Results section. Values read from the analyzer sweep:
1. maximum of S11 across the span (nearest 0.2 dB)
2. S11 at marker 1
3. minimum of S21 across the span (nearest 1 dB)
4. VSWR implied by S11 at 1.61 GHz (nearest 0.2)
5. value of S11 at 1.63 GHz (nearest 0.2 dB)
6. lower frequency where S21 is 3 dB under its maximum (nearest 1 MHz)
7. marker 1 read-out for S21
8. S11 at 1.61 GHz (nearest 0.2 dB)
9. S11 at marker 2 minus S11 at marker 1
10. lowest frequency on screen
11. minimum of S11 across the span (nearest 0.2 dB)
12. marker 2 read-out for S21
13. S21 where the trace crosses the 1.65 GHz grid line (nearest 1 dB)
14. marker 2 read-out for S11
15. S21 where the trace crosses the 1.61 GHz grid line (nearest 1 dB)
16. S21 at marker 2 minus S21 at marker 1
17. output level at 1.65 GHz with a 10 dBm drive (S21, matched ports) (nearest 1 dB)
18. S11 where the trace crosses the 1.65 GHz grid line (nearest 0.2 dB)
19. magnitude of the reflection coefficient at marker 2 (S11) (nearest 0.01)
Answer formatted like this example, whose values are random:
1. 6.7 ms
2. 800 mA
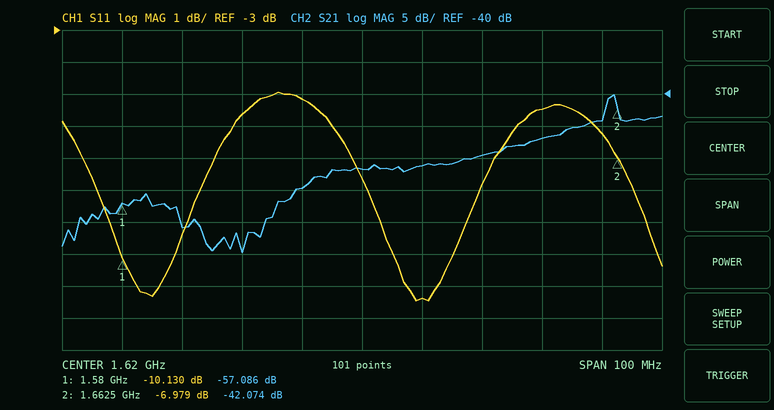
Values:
1. -5.0 dB
2. -10.130 dB
3. -65 dB
4. 3.4
5. -11.4 dB
6. 1.660 GHz
7. -57.086 dB
8. -5.2 dB
9. 3.151 dB
10. 1.57 GHz
11. -11.4 dB
12. -42.074 dB
13. -47 dB
14. -6.979 dB
15. -55 dB
16. 15.012 dB
17. -37 dBm
18. -5.4 dB
19. 0.45
